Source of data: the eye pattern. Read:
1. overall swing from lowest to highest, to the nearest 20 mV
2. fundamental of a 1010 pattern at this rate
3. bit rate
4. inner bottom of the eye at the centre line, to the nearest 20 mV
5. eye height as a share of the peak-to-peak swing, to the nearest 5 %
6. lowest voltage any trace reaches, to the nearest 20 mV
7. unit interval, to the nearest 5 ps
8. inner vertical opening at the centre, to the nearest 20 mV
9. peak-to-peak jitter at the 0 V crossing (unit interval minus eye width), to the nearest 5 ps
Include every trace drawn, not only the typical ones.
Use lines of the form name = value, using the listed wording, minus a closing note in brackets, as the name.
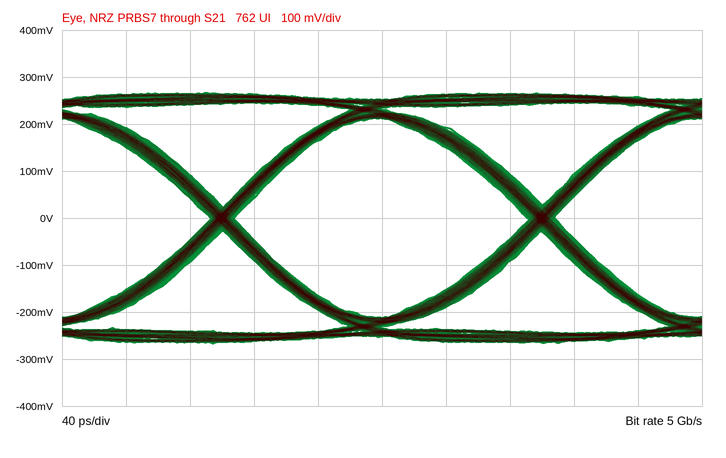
overall swing from lowest to highest, to the nearest 20 mV = 540 mV
fundamental of a 1010 pattern at this rate = 2.5 GHz
bit rate = 5 Gb/s
inner bottom of the eye at the centre line, to the nearest 20 mV = -220 mV
eye height as a share of the peak-to-peak swing, to the nearest 5 % = 80 %
lowest voltage any trace reaches, to the nearest 20 mV = -260 mV
unit interval, to the nearest 5 ps = 200 ps
inner vertical opening at the centre, to the nearest 20 mV = 420 mV
peak-to-peak jitter at the 0 V crossing (unit interval minus eye width), to the nearest 5 ps = 15 ps
